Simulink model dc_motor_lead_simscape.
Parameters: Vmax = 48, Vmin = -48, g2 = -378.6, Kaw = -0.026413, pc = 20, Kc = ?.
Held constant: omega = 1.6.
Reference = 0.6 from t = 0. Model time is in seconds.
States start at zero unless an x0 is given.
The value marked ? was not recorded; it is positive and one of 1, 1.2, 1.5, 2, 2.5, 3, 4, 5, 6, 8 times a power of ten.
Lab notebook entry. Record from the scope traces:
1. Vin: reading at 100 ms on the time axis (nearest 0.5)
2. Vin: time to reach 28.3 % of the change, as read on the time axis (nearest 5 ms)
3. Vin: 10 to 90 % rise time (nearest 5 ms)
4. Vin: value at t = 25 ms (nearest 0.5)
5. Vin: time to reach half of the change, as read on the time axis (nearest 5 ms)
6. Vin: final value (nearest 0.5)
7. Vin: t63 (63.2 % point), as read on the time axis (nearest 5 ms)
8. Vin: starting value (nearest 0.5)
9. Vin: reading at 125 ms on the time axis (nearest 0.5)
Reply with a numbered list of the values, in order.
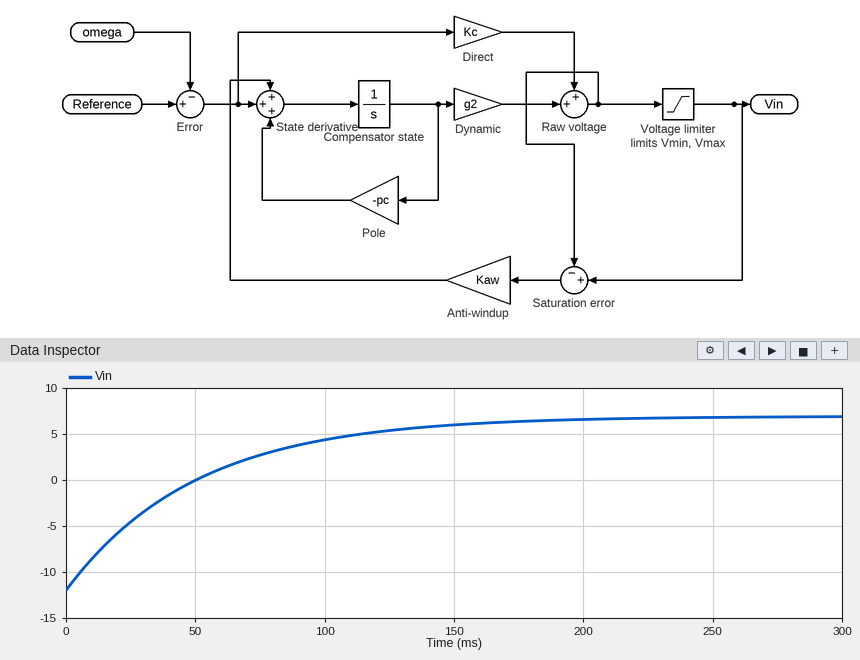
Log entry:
1. 4.5
2. 15 ms
3. 110 ms
4. -4.5
5. 35 ms
6. 7.0
7. 50 ms
8. -12.0
9. 5.5
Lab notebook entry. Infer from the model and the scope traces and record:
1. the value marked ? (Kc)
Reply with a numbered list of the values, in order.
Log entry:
1. 12
